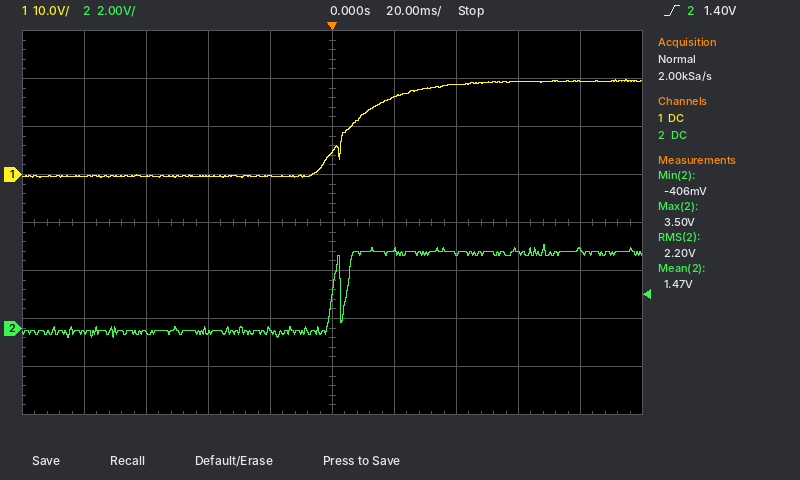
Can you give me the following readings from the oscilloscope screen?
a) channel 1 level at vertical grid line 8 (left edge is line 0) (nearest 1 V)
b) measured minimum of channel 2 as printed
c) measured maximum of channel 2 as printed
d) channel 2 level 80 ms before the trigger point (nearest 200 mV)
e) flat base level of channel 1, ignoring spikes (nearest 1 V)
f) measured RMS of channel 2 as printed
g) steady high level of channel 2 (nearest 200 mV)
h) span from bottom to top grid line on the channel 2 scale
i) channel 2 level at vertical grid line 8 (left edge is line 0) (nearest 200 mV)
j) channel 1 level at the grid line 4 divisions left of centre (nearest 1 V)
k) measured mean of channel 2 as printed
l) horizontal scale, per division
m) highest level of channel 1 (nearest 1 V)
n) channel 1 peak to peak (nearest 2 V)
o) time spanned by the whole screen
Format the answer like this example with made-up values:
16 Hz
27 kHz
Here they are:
19 V
-406 mV
3.50 V
-200 mV
0 V
2.20 V
3.2 V
16 V
3.2 V
0 V
1.47 V
20 ms
20 V
20 V
200 ms
